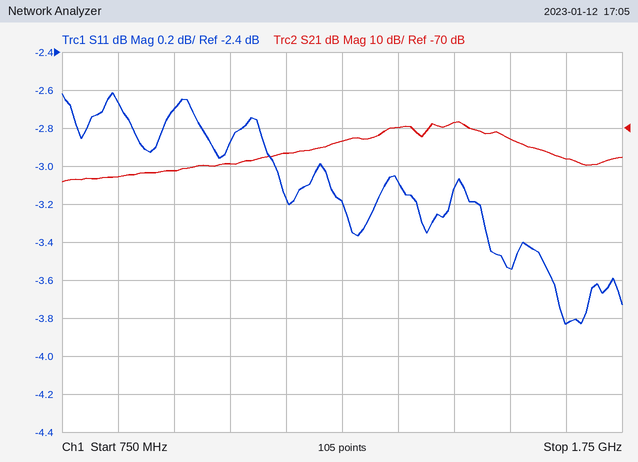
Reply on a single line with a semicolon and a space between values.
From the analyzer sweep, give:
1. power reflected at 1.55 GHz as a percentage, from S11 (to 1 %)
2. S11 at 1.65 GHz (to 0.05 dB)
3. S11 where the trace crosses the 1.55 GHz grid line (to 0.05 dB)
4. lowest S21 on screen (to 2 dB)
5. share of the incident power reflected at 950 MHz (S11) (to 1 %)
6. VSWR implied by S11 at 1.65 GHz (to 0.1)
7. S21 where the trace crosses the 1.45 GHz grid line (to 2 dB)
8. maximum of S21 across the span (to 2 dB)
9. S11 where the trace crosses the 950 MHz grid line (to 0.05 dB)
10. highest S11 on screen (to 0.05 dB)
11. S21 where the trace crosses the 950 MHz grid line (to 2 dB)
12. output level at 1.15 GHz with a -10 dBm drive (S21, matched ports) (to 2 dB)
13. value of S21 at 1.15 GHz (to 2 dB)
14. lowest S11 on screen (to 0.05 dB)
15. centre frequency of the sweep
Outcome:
44 %; -3.85 dB; -3.55 dB; -84 dB; 54 %; 4.6; -68 dB; -68 dB; -2.70 dB; -2.60 dB; -82 dB; -86 dBm; -76 dB; -3.85 dB; 1.25 GHz
